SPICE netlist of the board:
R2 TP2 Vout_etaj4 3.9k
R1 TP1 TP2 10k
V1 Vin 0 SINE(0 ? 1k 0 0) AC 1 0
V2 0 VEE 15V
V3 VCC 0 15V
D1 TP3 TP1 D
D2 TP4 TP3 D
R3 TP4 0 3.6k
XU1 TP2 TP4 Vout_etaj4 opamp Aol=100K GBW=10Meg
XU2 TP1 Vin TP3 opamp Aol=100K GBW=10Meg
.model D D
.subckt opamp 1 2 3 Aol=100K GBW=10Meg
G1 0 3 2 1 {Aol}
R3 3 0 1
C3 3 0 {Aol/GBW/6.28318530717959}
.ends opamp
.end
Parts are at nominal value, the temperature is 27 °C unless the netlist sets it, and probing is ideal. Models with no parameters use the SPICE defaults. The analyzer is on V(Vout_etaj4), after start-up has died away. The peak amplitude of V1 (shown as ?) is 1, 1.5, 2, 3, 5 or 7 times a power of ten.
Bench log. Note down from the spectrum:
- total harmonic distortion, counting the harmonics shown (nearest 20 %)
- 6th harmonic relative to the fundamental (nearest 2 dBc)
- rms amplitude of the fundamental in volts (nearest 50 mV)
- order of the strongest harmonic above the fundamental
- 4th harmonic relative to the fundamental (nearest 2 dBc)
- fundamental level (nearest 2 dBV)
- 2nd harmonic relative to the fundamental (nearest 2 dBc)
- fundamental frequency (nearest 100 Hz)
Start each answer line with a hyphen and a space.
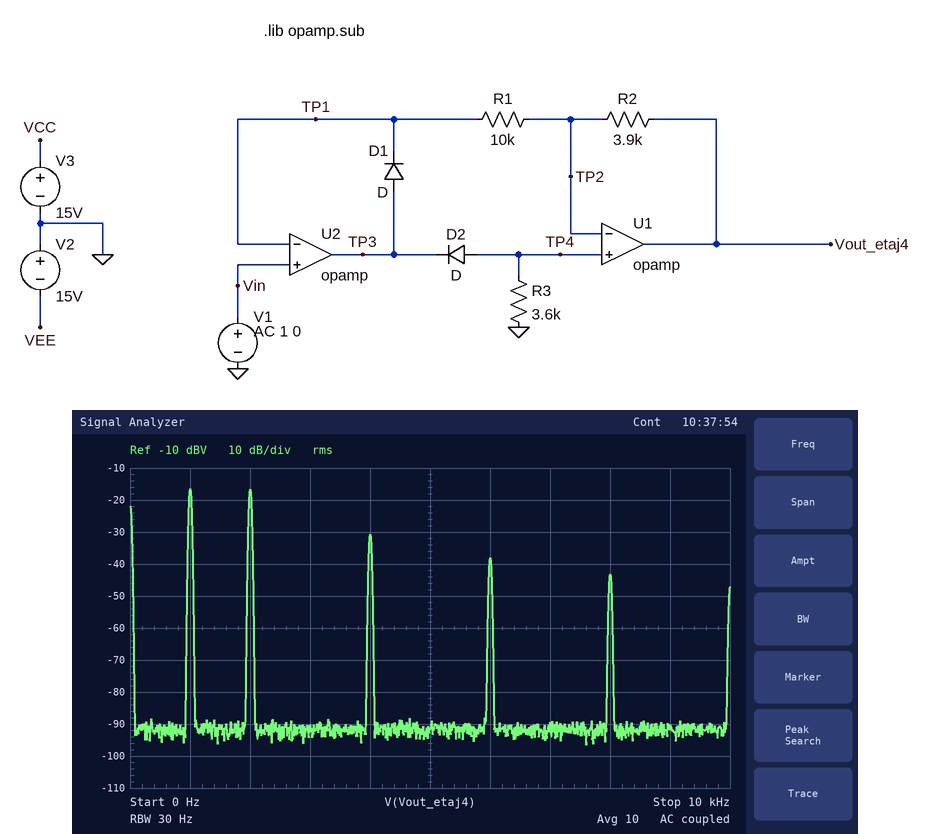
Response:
- 100 %
- -22 dBc
- 150 mV
- 2
- -14 dBc
- -16 dBV
- 0 dBc
- 1.0 kHz
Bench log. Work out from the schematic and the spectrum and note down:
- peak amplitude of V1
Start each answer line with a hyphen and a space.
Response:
- 700 mV
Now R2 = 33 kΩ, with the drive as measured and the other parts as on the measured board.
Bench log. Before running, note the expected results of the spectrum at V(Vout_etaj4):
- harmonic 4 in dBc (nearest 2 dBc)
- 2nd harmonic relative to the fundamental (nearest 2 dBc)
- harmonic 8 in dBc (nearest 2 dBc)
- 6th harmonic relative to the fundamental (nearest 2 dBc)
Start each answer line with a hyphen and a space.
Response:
- -16 dBc
- -2 dBc
- -28 dBc
- -24 dBc
